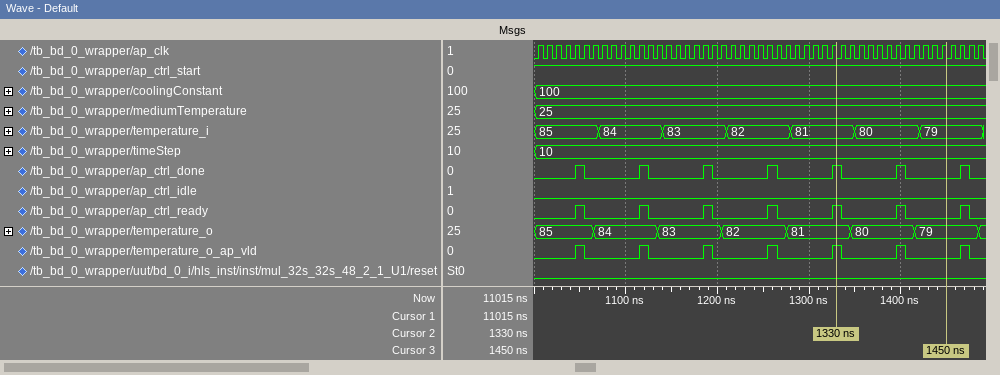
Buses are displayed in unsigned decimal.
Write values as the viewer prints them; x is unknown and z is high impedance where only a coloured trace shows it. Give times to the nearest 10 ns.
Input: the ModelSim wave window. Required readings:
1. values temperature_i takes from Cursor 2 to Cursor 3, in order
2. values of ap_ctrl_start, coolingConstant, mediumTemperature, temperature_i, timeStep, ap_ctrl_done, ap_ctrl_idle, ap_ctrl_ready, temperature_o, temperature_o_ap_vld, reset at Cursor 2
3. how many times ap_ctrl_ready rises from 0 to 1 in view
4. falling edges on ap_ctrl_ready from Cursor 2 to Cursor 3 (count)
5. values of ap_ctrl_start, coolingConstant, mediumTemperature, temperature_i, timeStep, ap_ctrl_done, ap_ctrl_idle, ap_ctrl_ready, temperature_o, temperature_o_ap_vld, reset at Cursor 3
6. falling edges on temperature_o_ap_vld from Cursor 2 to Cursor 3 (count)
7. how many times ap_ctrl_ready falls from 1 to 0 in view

81, 80, 79
ap_ctrl_start=1, coolingConstant=100, mediumTemperature=25, temperature_i=81, timeStep=10, ap_ctrl_done=1, ap_ctrl_idle=0, ap_ctrl_ready=1, temperature_o=81, temperature_o_ap_vld=1, reset=0
7
2
ap_ctrl_start=1, coolingConstant=100, mediumTemperature=25, temperature_i=79, timeStep=10, ap_ctrl_done=0, ap_ctrl_idle=0, ap_ctrl_ready=0, temperature_o=79, temperature_o_ap_vld=0, reset=0
2
7
